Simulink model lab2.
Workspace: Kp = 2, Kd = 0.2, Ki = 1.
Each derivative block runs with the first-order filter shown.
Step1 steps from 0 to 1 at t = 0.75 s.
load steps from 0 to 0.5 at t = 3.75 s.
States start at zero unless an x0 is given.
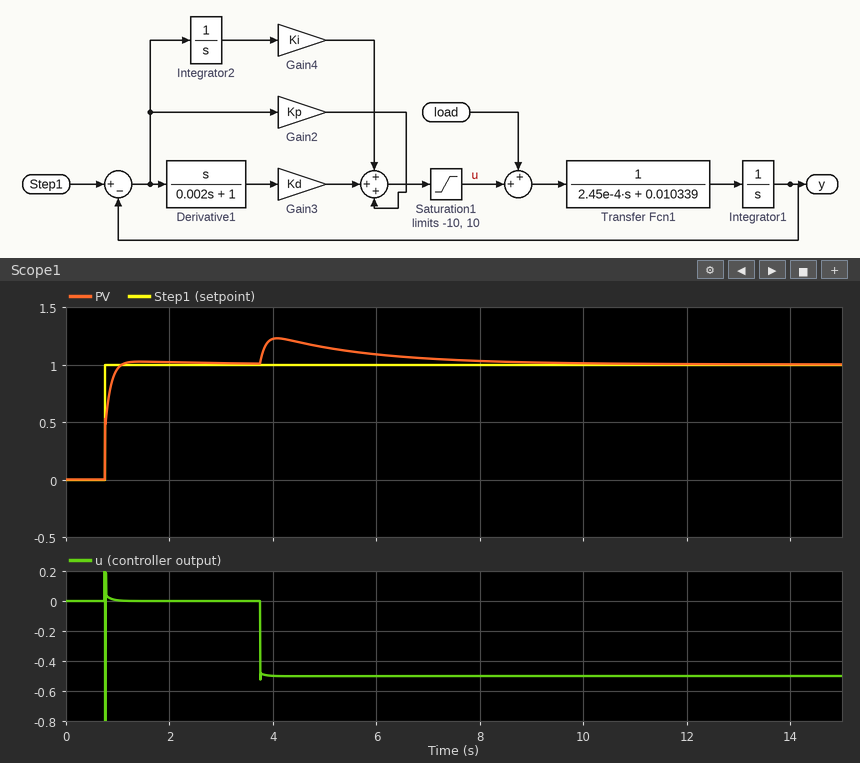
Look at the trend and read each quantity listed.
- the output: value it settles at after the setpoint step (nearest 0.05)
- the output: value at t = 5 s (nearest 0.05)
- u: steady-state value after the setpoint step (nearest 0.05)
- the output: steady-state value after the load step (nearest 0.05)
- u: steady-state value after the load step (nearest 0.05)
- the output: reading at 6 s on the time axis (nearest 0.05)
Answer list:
1.00
1.15
0.00
1.00
-0.50
1.10
